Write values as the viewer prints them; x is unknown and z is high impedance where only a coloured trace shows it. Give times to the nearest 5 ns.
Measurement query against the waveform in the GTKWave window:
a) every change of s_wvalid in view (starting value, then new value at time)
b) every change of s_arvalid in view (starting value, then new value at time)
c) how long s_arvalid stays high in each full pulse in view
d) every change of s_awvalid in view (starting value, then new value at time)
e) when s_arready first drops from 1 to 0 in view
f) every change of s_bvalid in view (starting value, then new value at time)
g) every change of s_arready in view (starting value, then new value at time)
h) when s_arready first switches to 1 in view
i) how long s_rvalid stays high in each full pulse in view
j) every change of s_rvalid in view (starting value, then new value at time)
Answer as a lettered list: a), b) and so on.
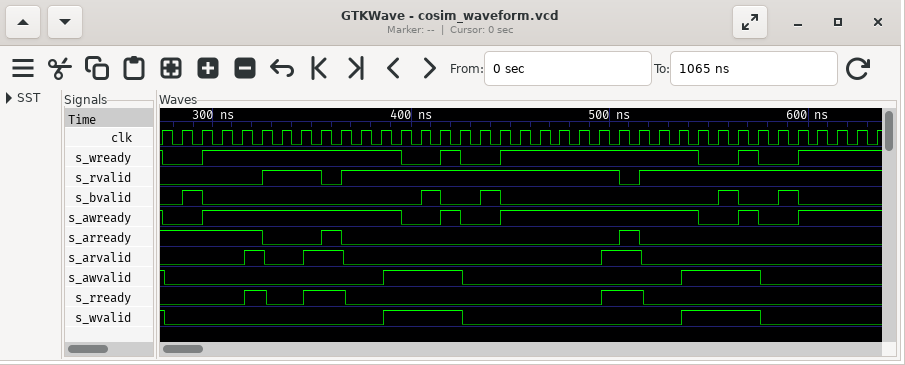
a) 1, 0 at 275 ns, 1 at 385 ns, 0 at 425 ns, 1 at 535 ns, 0 at 575 ns
b) 0, 1 at 315 ns, 0 at 325 ns, 1 at 345 ns, 0 at 365 ns, 1 at 495 ns, 0 at 515 ns
c) 10 ns, 20 ns, 20 ns
d) 1, 0 at 275 ns, 1 at 385 ns, 0 at 425 ns, 1 at 535 ns, 0 at 575 ns
e) 325 ns
f) 0, 1 at 285 ns, 0 at 295 ns, 1 at 405 ns, 0 at 415 ns, 1 at 435 ns, 0 at 445 ns, 1 at 555 ns, 0 at 565 ns, 1 at 585 ns, 0 at 595 ns
g) 1, 0 at 325 ns, 1 at 355 ns, 0 at 365 ns, 1 at 505 ns, 0 at 515 ns
h) 355 ns
i) 30 ns, 140 ns
j) 0, 1 at 325 ns, 0 at 355 ns, 1 at 365 ns, 0 at 505 ns, 1 at 515 ns
